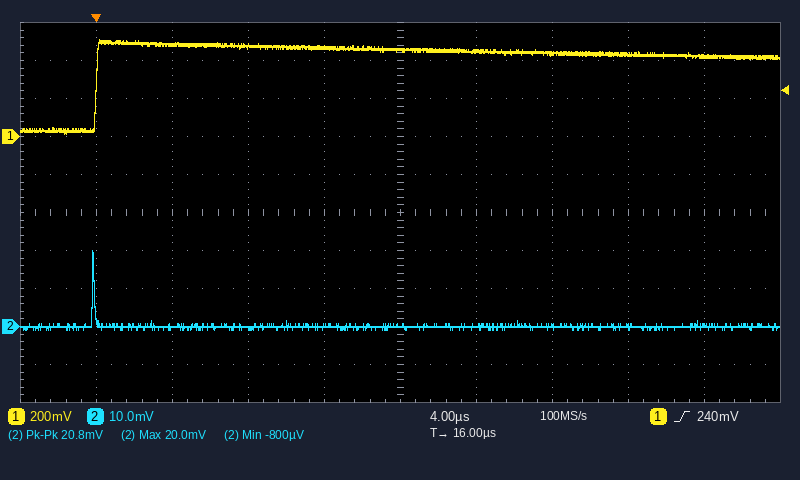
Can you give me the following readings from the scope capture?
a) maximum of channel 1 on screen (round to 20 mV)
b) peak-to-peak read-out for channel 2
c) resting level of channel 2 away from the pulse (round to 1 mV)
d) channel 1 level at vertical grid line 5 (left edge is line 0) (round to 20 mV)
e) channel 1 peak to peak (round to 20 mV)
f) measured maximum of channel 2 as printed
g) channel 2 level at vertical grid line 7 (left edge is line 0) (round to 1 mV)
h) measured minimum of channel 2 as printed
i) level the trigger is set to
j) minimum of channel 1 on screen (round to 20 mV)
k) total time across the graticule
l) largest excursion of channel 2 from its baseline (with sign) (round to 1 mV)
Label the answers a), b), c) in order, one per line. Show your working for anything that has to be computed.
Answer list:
a) 520 mV
b) 20.8 mV
c) 0 mV
d) 460 mV
e) 520 mV − (20 mV) = 500 mV
f) 20.0 mV
g) 0 mV
h) -800 µV
i) 240 mV
j) 20 mV
k) 40 µs
l) +20 mV
